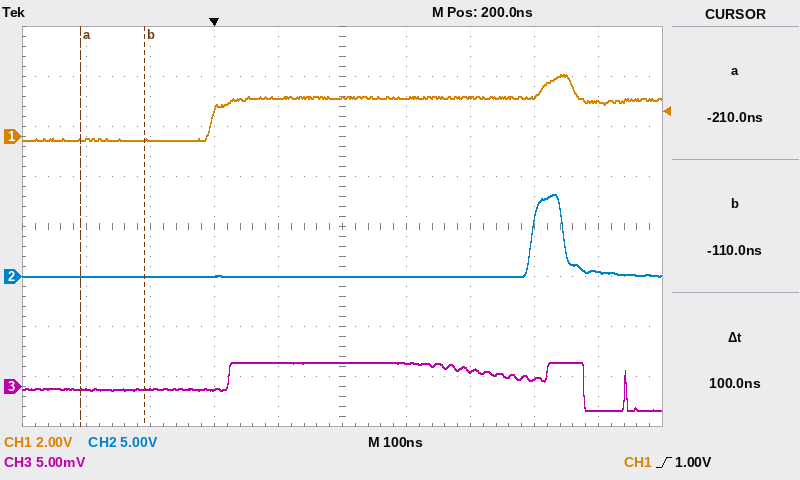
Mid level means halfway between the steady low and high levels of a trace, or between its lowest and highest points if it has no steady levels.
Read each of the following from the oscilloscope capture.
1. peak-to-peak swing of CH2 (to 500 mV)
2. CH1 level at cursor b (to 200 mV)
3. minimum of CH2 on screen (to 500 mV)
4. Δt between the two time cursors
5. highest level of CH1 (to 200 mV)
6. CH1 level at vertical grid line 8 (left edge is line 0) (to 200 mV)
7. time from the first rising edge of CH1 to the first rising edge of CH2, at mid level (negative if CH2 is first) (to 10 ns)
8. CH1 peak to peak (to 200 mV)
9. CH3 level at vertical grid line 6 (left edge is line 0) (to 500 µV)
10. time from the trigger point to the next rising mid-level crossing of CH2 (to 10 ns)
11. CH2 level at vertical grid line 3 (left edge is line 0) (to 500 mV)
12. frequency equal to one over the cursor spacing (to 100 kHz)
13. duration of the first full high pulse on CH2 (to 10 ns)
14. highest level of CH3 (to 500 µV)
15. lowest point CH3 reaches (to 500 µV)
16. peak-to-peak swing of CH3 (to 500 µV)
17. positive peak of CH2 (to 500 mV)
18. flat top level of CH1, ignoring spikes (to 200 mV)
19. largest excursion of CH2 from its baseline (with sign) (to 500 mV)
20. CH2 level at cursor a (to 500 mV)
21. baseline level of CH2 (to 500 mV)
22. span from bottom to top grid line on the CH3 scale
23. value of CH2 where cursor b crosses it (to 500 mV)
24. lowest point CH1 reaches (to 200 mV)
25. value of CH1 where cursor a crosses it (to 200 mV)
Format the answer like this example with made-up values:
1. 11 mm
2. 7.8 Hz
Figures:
1. 8.0 V
2. -200 mV
3. 0.0 V
4. 100 ns
5. 2.4 V
6. 1.6 V
7. +500 ns
8. 2.6 V
9. 2.5 mV
10. 500 ns
11. 0.0 V
12. 10.0 MHz
13. 50 ns
14. 2.5 mV
15. -2.5 mV
16. 5.0 mV
17. 8.0 V
18. 1.6 V
19. +8.0 V
20. 0.0 V
21. 0.0 V
22. 40 mV
23. 0.0 V
24. -200 mV
25. -200 mV
